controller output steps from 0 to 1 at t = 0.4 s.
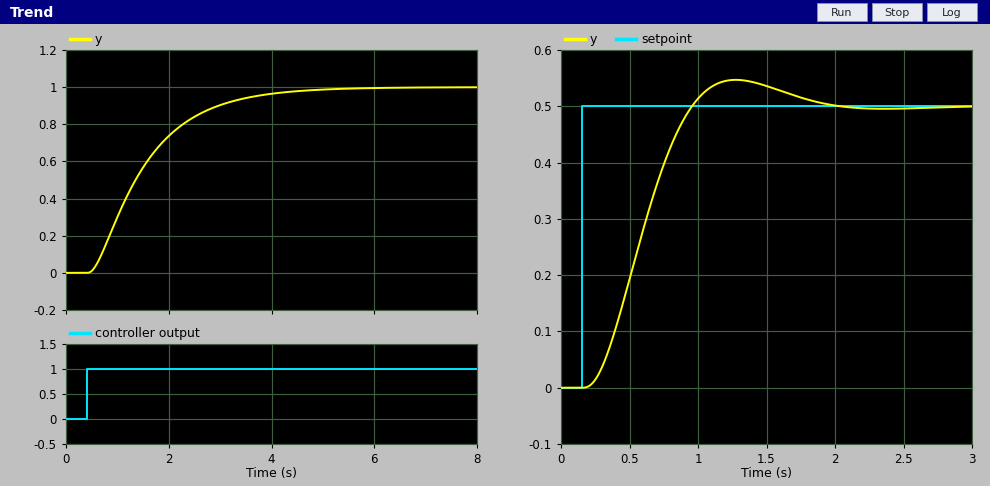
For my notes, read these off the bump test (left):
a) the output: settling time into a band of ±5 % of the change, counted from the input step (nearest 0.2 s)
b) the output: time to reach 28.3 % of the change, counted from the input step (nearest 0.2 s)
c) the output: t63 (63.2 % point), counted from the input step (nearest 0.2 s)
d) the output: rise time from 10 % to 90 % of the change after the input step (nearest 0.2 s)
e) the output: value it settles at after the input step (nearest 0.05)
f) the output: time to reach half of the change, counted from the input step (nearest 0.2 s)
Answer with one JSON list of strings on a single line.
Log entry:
["3.2 s", "0.6 s", "1.2 s", "2.2 s", "1.00", "1.0 s"]
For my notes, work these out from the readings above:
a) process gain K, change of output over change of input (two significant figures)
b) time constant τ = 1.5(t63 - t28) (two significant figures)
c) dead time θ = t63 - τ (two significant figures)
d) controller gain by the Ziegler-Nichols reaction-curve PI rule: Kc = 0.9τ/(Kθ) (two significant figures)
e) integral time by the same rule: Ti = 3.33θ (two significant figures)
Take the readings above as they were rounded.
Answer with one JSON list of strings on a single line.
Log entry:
["1.0", "0.90 s", "0.30 s", "2.7", "1.00 s"]
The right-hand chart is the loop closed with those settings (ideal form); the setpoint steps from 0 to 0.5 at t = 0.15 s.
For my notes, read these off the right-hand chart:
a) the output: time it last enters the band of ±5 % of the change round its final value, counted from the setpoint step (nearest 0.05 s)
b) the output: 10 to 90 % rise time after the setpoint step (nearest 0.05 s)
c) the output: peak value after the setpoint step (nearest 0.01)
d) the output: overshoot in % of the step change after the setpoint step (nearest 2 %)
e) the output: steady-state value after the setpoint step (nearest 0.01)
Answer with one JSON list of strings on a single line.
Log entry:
["1.50 s", "0.50 s", "0.55", "10 %", "0.50"]
